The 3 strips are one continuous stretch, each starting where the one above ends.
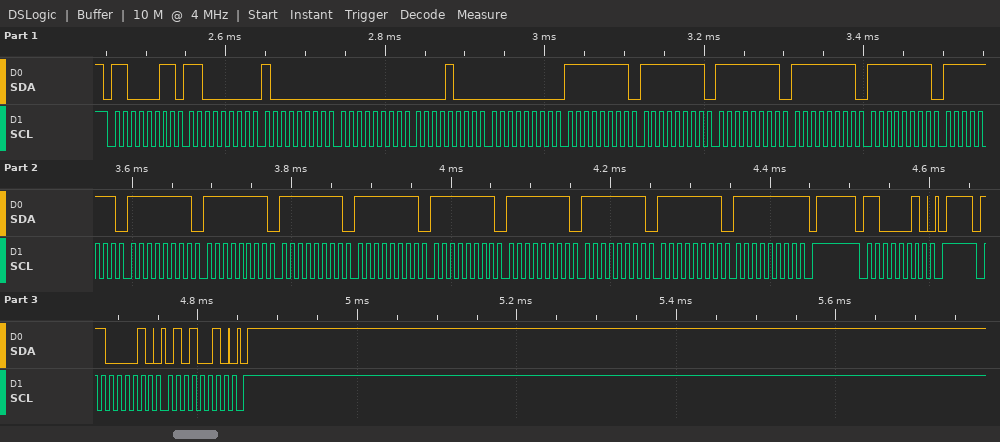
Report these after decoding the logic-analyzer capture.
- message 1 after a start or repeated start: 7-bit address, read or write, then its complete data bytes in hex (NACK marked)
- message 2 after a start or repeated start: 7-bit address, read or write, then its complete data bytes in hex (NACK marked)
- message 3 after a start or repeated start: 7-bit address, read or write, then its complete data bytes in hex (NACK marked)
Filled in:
0x61 read: C0 80 00 08 00 FF FF FF FF FF FF FF FF FF FF FF FF FF FF FF NACK
0x61 write
0x61 write: 52
